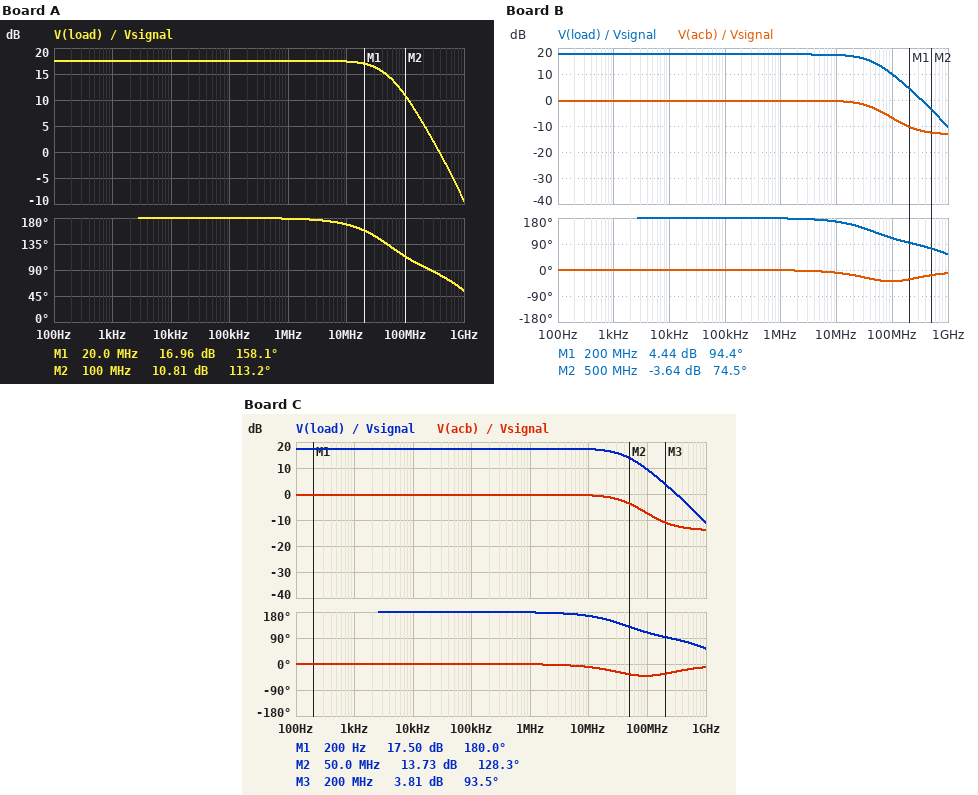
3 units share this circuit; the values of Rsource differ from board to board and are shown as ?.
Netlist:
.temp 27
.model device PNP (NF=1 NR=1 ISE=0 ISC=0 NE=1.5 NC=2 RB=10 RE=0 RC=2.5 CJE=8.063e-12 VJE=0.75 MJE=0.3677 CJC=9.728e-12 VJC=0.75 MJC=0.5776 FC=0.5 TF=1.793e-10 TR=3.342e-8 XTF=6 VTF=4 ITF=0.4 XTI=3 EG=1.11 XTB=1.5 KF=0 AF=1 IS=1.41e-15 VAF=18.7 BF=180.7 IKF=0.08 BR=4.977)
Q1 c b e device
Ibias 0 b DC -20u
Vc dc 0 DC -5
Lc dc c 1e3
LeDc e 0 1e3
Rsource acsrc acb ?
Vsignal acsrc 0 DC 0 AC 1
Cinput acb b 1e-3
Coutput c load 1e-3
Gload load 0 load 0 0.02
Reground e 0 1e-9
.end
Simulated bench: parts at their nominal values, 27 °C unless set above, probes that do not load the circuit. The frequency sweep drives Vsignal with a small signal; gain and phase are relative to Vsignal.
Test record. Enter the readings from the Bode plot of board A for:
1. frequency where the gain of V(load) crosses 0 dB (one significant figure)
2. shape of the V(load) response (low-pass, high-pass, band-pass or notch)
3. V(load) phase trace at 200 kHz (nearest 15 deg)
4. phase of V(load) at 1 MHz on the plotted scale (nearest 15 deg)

400 MHz
low-pass
180 deg
180 deg
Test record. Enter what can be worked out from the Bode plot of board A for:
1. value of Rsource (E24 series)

33 Ω
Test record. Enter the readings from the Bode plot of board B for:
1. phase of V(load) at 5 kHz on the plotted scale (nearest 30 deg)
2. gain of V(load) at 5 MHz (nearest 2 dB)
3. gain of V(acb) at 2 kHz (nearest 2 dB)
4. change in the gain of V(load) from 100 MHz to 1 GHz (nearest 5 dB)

180 deg
18 dB
0 dB
-20 dB
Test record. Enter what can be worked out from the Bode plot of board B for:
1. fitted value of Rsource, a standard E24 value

39 Ω
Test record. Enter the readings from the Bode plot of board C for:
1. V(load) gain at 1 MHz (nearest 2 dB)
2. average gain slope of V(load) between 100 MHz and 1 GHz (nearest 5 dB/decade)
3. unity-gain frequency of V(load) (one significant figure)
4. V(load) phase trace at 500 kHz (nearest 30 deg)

18 dB
-20 dB/decade
300 MHz
180 deg
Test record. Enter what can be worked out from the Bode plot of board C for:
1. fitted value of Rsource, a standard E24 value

43 Ω
